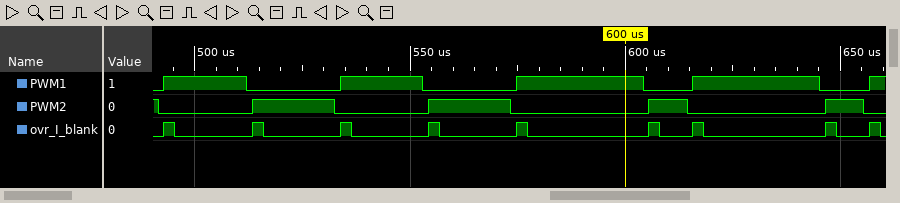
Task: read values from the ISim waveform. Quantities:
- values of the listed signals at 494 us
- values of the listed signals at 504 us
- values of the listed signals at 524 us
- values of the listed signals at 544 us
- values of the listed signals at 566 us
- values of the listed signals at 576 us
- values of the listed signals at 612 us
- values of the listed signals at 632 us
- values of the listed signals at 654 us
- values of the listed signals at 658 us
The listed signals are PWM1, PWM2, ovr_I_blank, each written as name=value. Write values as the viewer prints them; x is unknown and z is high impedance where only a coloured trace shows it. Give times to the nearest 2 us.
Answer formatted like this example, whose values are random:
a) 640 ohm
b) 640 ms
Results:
a) PWM1=1, PWM2=0, ovr_I_blank=1
b) PWM1=1, PWM2=0, ovr_I_blank=0
c) PWM1=0, PWM2=1, ovr_I_blank=0
d) PWM1=1, PWM2=0, ovr_I_blank=0
e) PWM1=0, PWM2=1, ovr_I_blank=0
f) PWM1=1, PWM2=0, ovr_I_blank=1
g) PWM1=0, PWM2=1, ovr_I_blank=0
h) PWM1=1, PWM2=0, ovr_I_blank=0
i) PWM1=0, PWM2=1, ovr_I_blank=0
j) PWM1=1, PWM2=0, ovr_I_blank=1
